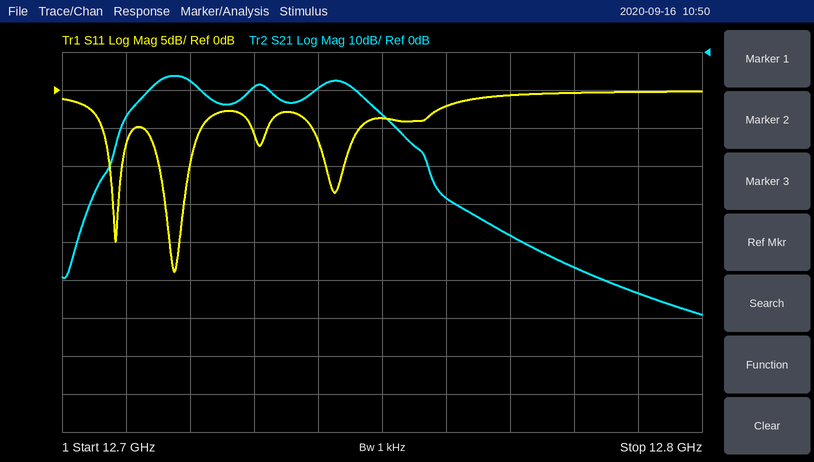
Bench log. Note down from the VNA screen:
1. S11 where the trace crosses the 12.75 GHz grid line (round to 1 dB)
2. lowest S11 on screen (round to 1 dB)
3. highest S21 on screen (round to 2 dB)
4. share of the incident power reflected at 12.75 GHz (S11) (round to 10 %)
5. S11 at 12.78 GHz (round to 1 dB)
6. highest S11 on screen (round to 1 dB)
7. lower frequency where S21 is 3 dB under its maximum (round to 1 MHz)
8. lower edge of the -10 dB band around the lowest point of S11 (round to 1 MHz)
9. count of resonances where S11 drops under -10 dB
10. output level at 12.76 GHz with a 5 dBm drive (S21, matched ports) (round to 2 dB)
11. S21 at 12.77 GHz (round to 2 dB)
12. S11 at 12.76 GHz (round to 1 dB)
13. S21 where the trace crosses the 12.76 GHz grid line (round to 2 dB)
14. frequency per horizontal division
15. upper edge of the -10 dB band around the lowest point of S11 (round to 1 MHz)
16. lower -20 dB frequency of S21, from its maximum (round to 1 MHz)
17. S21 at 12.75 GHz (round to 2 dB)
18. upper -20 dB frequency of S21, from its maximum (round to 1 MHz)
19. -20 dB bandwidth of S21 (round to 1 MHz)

-4 dB
-24 dB
-6 dB
40 %
0 dB
0 dB
12.714 GHz
12.715 GHz
3
-34 dBm
-48 dB
-2 dB
-38 dB
10 MHz
12.720 GHz
12.708 GHz
-16 dB
12.756 GHz
48 MHz
